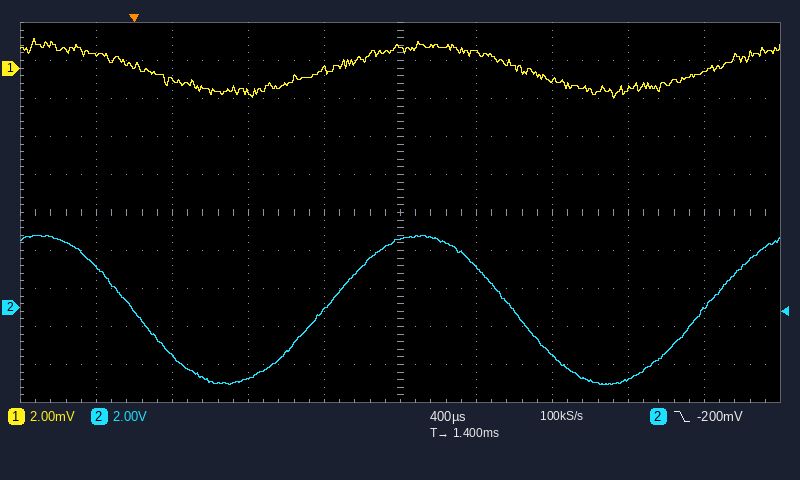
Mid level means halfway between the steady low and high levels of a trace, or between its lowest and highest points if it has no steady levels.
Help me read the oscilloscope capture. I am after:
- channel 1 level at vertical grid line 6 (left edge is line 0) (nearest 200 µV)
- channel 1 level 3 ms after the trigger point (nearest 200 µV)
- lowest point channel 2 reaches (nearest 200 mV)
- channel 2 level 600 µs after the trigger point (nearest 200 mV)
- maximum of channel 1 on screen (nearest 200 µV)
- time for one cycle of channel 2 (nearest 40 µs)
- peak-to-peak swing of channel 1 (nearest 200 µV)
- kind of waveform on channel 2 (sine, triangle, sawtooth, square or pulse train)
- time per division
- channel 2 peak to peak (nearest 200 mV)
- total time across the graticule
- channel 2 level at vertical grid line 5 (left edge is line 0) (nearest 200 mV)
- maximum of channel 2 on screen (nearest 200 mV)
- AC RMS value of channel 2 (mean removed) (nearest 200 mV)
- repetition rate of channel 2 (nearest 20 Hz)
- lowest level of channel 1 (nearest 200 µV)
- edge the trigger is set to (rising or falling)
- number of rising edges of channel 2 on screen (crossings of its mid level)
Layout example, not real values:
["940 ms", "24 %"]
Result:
["800 µV", "-200 µV", "-4.0 V", "-3.8 V", "1.6 mV", "2.00 ms", "3.2 mV", "sine", "400 µs", "7.8 V", "4 ms", "3.6 V", "3.8 V", "2.8 V", "500 Hz", "-1.6 mV", "falling", "2"]
